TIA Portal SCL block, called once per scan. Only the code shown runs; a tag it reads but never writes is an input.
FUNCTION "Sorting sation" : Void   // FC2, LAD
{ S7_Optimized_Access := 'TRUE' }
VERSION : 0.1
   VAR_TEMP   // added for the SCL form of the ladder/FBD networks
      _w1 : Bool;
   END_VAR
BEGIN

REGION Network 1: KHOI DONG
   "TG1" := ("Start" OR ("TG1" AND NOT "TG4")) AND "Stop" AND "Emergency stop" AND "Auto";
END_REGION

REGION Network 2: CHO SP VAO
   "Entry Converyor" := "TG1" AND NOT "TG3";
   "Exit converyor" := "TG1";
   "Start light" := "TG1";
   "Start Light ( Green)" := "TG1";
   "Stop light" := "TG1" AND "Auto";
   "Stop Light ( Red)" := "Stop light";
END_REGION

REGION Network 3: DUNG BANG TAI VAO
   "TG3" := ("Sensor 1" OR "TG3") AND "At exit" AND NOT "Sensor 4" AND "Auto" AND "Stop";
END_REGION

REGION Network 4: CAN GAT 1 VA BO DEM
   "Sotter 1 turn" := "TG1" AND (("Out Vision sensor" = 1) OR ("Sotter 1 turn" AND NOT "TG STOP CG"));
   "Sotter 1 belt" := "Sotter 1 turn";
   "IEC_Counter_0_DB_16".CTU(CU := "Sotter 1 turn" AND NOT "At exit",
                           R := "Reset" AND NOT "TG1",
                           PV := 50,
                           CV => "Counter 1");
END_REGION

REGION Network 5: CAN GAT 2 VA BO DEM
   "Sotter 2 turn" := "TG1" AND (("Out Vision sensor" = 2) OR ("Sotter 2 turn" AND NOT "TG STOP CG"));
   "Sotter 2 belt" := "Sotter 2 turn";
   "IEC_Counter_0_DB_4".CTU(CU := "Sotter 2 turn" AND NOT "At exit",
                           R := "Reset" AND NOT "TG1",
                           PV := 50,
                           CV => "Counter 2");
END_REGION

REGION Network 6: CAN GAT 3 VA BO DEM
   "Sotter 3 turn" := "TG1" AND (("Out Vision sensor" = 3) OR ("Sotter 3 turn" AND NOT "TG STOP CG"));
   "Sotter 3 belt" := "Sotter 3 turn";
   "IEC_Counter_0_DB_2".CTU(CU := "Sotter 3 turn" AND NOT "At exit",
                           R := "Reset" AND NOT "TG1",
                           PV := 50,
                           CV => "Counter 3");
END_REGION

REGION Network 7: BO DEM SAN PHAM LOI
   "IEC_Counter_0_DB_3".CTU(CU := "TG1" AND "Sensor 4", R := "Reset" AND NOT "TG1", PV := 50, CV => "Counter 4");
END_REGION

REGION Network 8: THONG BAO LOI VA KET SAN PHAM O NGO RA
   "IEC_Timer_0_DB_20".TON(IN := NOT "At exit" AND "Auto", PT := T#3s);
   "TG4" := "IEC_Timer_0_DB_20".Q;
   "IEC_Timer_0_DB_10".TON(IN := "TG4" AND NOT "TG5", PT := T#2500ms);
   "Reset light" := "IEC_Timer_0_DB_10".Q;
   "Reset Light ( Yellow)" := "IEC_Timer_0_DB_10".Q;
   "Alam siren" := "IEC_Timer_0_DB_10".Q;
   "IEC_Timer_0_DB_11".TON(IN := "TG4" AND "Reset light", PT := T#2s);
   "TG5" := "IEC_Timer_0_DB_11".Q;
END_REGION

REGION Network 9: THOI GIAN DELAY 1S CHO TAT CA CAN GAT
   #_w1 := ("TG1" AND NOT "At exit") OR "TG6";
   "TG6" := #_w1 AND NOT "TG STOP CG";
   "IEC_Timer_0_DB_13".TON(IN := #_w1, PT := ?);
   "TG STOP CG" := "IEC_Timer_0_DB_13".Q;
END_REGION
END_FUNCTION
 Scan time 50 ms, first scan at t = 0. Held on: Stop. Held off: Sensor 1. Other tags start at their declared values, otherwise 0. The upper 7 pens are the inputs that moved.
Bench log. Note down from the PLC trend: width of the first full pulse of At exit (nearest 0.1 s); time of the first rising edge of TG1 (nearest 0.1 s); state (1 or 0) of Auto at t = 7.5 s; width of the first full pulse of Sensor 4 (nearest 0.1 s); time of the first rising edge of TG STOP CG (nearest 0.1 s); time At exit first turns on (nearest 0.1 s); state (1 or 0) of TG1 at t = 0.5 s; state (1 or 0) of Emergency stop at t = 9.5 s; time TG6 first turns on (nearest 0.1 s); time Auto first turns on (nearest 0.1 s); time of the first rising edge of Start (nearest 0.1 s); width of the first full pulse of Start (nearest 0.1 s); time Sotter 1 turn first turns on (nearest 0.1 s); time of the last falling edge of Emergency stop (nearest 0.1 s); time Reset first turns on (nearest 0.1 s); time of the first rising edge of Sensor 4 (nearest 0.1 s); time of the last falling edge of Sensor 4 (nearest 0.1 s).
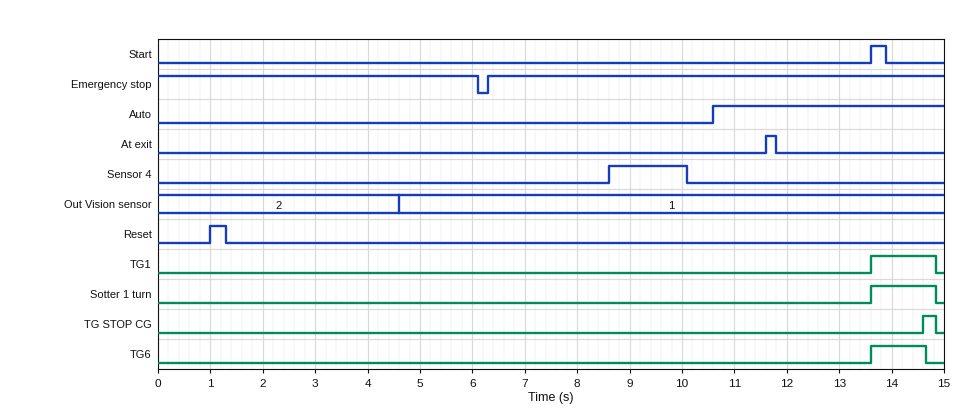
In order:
0.2 s
13.6 s
0
1.5 s
14.6 s
11.6 s
0
1
13.6 s
10.6 s
13.6 s
0.3 s
13.6 s
6.1 s
1.0 s
8.6 s
10.1 s
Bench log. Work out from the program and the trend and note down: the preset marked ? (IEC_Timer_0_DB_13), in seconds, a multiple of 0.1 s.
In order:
1.0 s
